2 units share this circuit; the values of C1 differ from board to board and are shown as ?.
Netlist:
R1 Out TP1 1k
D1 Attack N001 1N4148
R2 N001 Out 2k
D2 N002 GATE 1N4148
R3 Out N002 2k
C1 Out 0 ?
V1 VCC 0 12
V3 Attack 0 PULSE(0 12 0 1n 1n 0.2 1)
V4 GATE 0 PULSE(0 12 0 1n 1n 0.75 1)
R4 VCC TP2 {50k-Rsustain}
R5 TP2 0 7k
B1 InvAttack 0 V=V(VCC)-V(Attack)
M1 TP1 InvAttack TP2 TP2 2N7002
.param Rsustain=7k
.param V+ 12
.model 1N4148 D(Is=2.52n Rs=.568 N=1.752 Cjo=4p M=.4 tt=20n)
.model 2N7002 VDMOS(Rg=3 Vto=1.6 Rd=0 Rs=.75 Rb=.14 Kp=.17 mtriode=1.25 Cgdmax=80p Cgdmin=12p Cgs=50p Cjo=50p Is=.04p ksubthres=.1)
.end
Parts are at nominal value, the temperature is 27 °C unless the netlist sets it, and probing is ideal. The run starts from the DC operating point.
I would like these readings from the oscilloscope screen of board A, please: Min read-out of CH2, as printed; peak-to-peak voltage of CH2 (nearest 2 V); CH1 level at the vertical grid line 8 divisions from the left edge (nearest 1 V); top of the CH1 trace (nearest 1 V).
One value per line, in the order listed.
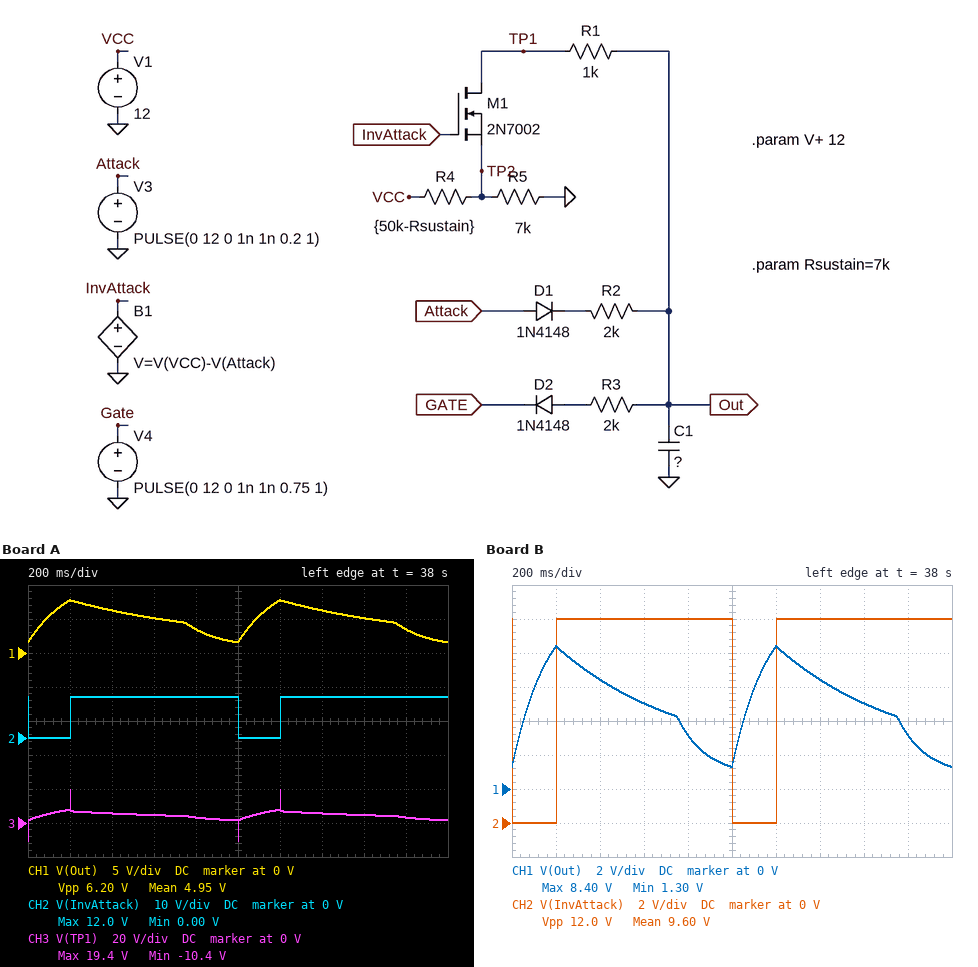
0.00 V
12 V
5 V
8 V
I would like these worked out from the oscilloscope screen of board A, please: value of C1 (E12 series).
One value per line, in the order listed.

100 µF
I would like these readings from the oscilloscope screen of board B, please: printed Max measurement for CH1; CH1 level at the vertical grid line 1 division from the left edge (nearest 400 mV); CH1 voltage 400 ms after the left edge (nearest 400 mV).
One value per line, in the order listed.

8.40 V
8.4 V
6.4 V
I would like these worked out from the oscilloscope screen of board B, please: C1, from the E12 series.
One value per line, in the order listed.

82 µF
